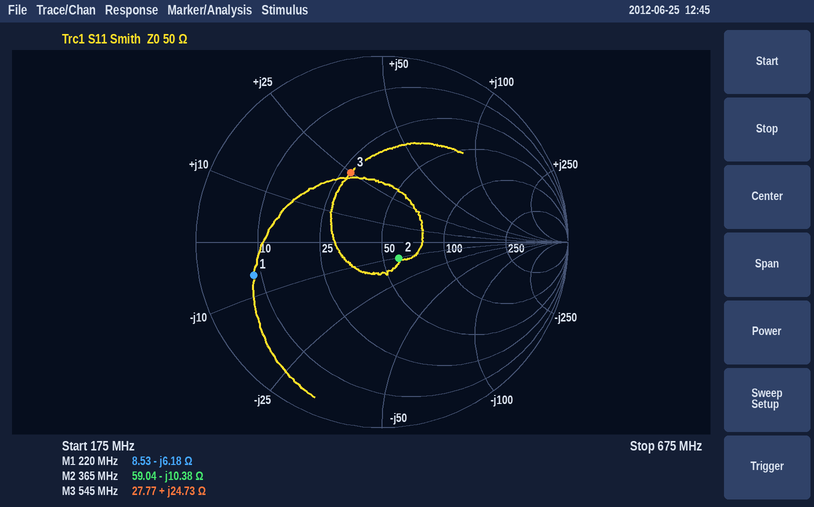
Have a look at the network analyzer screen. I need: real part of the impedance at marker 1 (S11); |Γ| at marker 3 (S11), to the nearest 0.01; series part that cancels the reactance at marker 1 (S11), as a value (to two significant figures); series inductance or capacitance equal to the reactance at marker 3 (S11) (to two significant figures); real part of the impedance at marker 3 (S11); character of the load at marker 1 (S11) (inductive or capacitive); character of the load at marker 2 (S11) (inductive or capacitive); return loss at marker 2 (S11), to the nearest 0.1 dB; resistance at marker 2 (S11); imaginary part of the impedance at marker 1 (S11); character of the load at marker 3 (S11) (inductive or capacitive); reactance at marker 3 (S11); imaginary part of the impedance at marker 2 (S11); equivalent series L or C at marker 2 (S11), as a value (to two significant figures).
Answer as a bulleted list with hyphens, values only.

- 8.53 Ω
- 0.41
- 4.5 nH
- 7.2 nH
- 27.77 Ω
- capacitive
- capacitive
- 18.0 dB
- 59.04 Ω
- -6.18 Ω
- inductive
- +24.73 Ω
- -10.38 Ω
- 42 pF
